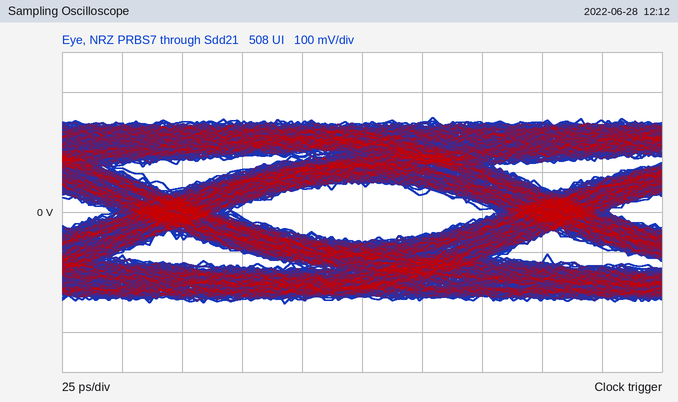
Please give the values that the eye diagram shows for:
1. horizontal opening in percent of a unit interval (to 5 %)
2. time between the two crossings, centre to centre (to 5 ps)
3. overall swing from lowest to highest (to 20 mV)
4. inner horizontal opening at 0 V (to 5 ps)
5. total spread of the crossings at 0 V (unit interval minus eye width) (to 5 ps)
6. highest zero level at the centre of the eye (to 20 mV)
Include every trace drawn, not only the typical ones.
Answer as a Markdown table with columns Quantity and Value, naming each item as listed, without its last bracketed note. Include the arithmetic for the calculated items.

| Quantity | Value |
|---|---|
| horizontal opening in percent of a unit interval | 110 ps / 160 ps ≈ 68.8 %, so 70 % to the nearest 5 % |
| time between the two crossings, centre to centre | 160 ps |
| overall swing from lowest to highest | 460 mV |
| inner horizontal opening at 0 V | 110 ps |
| total spread of the crossings at 0 V (unit interval minus eye width) | 50 ps |
| highest zero level at the centre of the eye | -80 mV |
